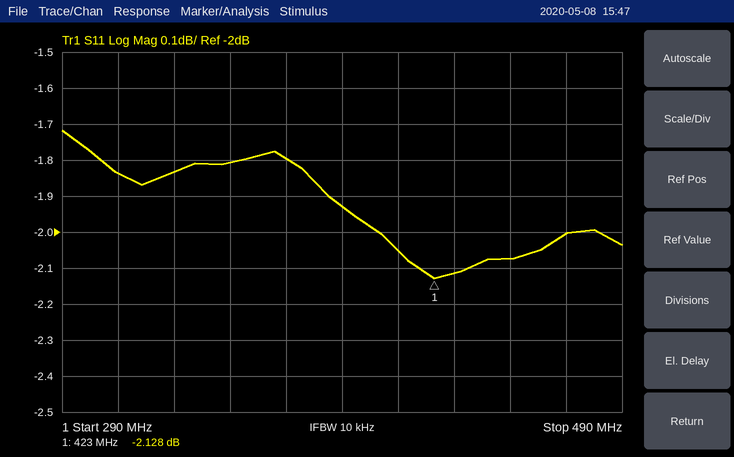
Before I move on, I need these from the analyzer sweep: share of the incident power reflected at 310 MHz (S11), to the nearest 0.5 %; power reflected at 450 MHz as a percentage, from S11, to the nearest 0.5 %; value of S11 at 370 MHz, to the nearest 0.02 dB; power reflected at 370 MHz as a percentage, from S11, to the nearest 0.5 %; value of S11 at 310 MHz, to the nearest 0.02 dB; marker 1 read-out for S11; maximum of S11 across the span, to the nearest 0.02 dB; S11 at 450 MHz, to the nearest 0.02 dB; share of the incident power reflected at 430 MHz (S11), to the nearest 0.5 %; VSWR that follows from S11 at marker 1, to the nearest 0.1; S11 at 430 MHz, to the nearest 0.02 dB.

65.5 %
62.0 %
-1.80 dB
66.0 %
-1.84 dB
-2.128 dB
-1.72 dB
-2.08 dB
61.5 %
8.2
-2.12 dB
